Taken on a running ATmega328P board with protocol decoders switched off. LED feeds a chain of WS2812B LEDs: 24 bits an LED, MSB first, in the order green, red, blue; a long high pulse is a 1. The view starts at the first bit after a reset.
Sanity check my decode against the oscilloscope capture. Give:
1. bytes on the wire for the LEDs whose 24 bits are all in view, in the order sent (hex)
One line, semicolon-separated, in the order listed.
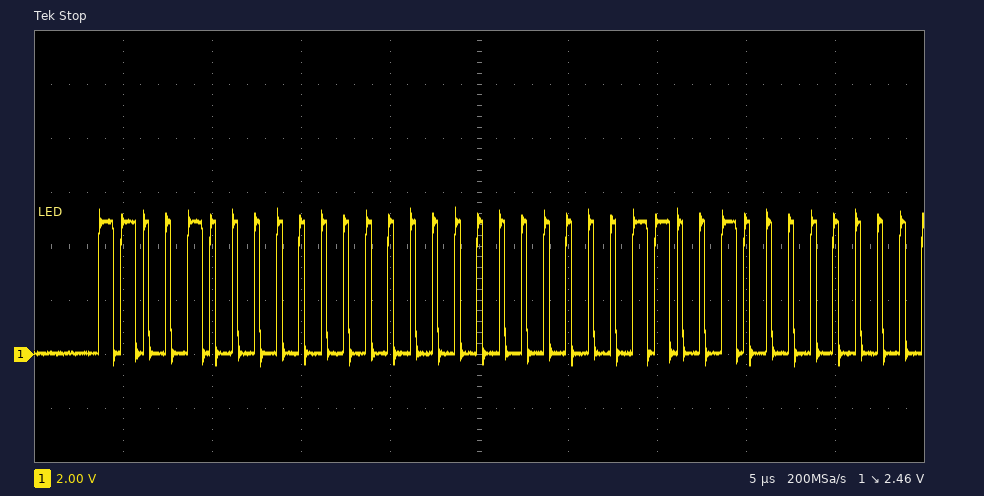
C8 00 00
